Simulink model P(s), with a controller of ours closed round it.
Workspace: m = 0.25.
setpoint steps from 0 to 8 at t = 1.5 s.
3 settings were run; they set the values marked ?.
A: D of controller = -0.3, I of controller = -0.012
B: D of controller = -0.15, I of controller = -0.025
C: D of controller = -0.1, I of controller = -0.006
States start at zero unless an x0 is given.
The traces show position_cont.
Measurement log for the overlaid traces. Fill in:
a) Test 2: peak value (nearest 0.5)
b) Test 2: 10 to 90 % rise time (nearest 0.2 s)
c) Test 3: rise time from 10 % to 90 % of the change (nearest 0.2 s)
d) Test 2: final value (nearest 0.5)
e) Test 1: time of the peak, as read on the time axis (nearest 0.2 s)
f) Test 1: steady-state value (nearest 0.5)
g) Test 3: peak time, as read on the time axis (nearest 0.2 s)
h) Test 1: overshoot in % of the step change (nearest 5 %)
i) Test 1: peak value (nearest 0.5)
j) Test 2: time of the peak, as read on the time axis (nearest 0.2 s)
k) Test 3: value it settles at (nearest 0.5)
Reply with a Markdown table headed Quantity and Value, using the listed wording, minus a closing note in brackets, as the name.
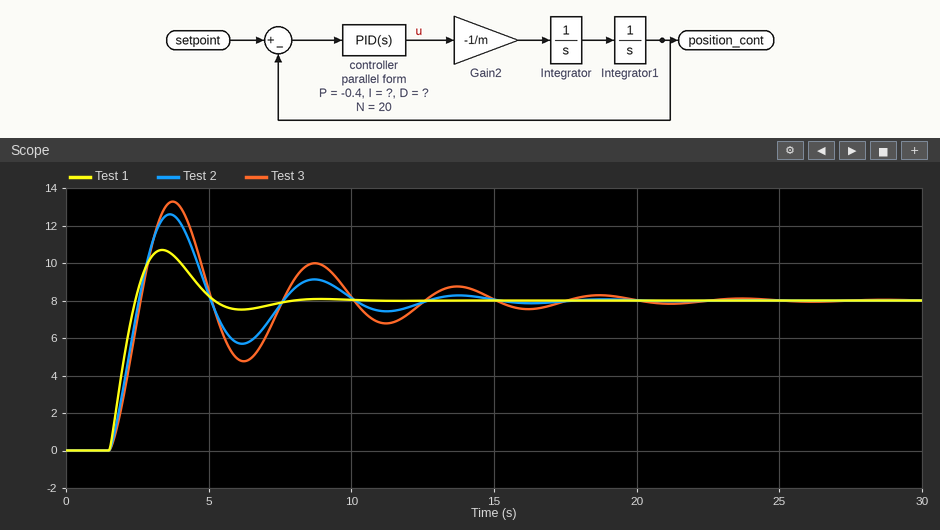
| Quantity | Value |
|---|---|
| Test 2: peak value | 12.5 |
| Test 2: 10 to 90 % rise time | 0.8 s |
| Test 3: rise time from 10 % to 90 % of the change | 0.8 s |
| Test 2: final value | 8.0 |
| Test 1: time of the peak, as read on the time axis | 3.4 s |
| Test 1: steady-state value | 8.0 |
| Test 3: peak time, as read on the time axis | 3.8 s |
| Test 1: overshoot in % of the step change | 35 % |
| Test 1: peak value | 10.5 |
| Test 2: time of the peak, as read on the time axis | 3.6 s |
| Test 3: value it settles at | 8.0 |
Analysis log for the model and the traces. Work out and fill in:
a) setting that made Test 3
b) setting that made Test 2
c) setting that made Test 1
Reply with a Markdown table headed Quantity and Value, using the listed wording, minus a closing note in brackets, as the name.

| Quantity | Value |
|---|---|
| setting that made Test 3 | C |
| setting that made Test 2 | B |
| setting that made Test 1 | A |
